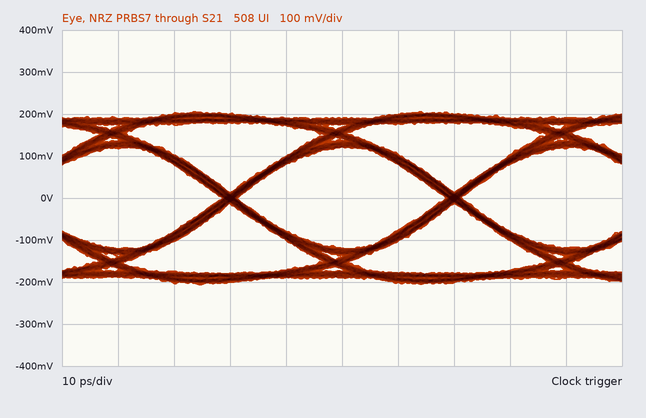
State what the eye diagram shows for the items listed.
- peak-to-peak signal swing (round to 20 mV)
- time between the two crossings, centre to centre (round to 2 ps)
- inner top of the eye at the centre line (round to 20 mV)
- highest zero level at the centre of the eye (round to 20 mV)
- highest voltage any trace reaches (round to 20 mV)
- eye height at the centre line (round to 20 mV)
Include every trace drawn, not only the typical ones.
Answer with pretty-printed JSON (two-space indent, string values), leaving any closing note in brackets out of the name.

{
  "peak-to-peak signal swing": "420 mV",
  "time between the two crossings, centre to centre": "40 ps",
  "inner top of the eye at the centre line": "120 mV",
  "highest zero level at the centre of the eye": "-120 mV",
  "highest voltage any trace reaches": "200 mV",
  "eye height at the centre line": "240 mV"
}
